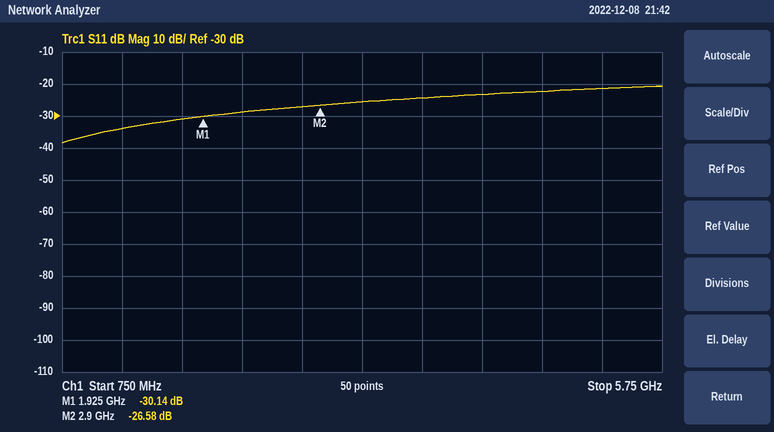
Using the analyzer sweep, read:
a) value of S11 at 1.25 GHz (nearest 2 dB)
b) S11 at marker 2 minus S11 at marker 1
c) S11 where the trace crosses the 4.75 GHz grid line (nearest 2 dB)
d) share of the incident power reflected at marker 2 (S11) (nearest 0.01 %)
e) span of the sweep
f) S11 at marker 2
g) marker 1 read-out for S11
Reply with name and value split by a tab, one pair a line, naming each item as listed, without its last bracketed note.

value of S11 at 1.25 GHz	-34 dB
S11 at marker 2 minus S11 at marker 1	3.56 dB
S11 where the trace crosses the 4.75 GHz grid line	-22 dB
share of the incident power reflected at marker 2 (S11)	0.22 %
span of the sweep	5 GHz
S11 at marker 2	-26.58 dB
marker 1 read-out for S11	-30.14 dB
